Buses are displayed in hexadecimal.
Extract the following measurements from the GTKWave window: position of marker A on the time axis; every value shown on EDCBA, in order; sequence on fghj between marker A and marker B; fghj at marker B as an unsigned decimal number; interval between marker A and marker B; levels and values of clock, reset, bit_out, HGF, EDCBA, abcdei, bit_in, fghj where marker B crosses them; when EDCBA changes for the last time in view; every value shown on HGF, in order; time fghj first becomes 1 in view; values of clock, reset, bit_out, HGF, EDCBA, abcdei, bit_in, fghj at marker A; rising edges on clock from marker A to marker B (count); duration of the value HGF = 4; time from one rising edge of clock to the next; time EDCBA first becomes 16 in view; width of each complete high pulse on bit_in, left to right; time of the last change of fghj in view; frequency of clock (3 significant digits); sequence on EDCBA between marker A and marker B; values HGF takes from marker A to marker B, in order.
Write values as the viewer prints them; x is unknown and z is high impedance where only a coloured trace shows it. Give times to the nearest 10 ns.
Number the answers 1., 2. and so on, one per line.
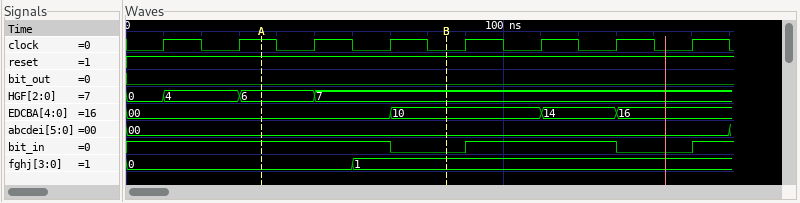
1. 40 ns
2. 00, 10, 14, 16
3. 0, 1
4. 1
5. 50 ns
6. clock=0, reset=1, bit_out=0, HGF=7, EDCBA=10, abcdei=00, bit_in=0, fghj=1
7. 130 ns
8. 0, 4, 6, 7
9. 60 ns
10. clock=1, reset=1, bit_out=0, HGF=6, EDCBA=00, abcdei=00, bit_in=1, fghj=0
11. 2
12. 20 ns
13. 20 ns
14. 130 ns
15. 40 ns
16. 60 ns
17. 50.0 MHz
18. 00, 10
19. 6, 7
